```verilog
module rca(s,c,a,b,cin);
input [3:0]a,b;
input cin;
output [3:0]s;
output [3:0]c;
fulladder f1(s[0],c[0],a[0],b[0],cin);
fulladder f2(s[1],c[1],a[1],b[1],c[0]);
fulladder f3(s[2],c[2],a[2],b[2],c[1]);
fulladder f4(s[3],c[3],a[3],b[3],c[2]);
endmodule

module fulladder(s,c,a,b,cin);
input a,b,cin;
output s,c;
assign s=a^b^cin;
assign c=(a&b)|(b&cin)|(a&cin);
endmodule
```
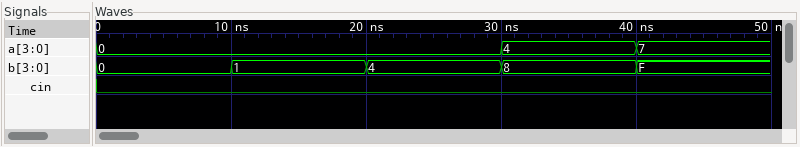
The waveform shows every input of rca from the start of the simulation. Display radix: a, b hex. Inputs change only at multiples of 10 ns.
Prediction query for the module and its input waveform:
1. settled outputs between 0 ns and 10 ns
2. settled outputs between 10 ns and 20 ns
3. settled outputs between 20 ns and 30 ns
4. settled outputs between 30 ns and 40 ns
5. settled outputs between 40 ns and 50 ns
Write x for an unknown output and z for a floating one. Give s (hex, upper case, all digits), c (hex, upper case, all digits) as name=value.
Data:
s=0, c=0
s=1, c=0
s=4, c=0
s=C, c=0
s=6, c=F
